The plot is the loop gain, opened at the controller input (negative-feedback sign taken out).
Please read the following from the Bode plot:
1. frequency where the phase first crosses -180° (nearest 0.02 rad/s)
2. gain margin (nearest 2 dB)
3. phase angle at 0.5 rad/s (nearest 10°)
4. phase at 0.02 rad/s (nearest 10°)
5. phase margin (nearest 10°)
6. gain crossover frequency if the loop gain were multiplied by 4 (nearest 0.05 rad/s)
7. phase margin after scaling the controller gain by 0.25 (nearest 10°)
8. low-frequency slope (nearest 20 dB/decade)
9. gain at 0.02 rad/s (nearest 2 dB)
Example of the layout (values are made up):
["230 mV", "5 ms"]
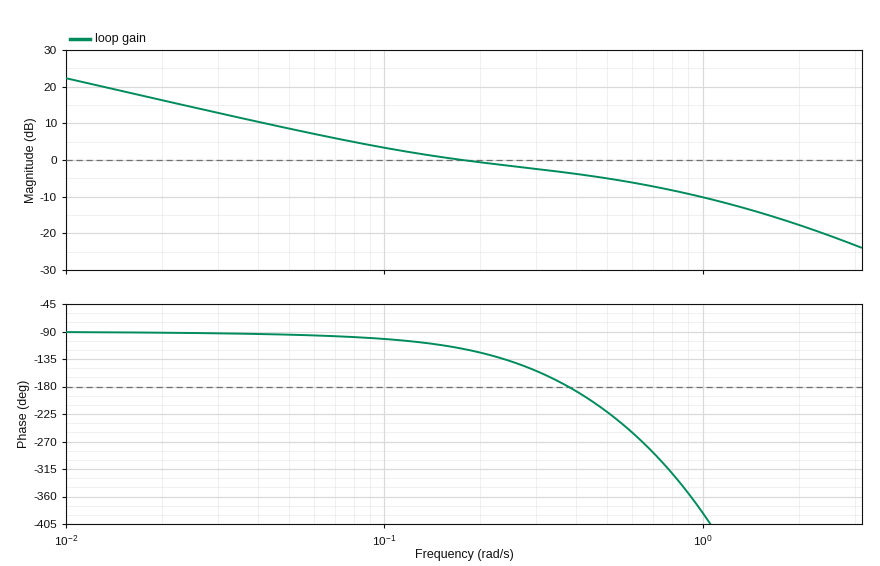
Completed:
["0.38 rad/s", "4 dB", "-220°", "-90°", "60°", "1.20 rad/s", "90°", "-20 dB/decade", "16 dB"]
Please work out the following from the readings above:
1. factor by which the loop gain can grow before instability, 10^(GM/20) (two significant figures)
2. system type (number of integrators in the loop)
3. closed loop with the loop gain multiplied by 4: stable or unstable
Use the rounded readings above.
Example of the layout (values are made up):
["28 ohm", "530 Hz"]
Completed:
["1.6", "1", "unstable"]
